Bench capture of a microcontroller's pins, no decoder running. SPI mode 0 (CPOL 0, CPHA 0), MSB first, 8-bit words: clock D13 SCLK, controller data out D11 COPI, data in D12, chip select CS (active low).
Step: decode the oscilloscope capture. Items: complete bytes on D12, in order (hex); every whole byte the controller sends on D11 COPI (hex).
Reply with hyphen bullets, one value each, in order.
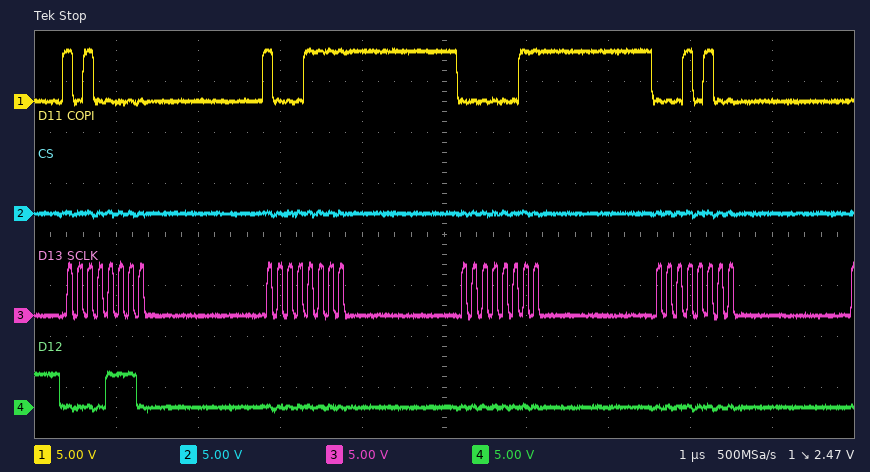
- 0x0E 0x00 0x00 0x00
- 0xA0 0x8F 0x03 0x14
